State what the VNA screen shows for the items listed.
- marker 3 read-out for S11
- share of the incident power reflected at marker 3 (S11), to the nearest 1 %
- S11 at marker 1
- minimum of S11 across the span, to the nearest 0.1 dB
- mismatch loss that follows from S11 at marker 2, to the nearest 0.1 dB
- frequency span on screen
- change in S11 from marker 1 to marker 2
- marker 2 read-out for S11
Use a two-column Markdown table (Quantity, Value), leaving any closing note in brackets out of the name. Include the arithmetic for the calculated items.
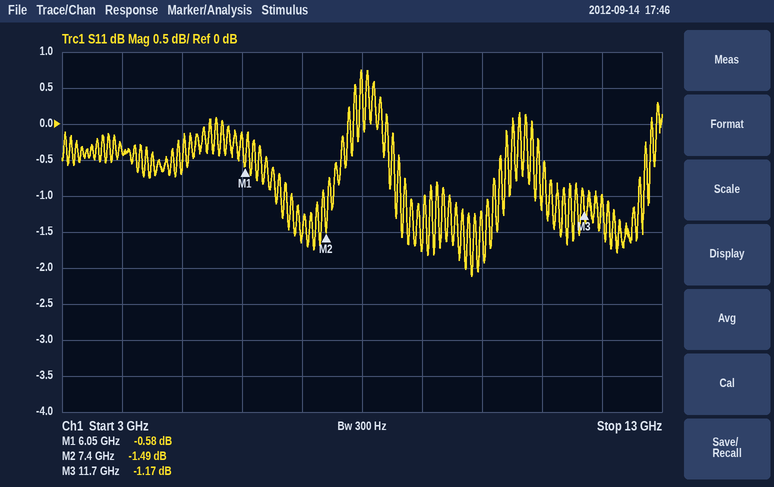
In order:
| Quantity | Value |
|---|---|
| marker 3 read-out for S11 | -1.17 dB |
| share of the incident power reflected at marker 3 (S11), to the nearest 1 % | 10^(-1.17/10) ≈ 76 % |
| S11 at marker 1 | -0.58 dB |
| minimum of S11 across the span, to the nearest 0.1 dB | -2.1 dB |
| mismatch loss that follows from S11 at marker 2, to the nearest 0.1 dB | −10 log10(1 − 10^(-1.49/10)) ≈ 5.4 dB |
| frequency span on screen | 10 GHz |
| change in S11 from marker 1 to marker 2 | -1.49 − (-0.58) = -0.91 dB |
| marker 2 read-out for S11 | -1.49 dB |
